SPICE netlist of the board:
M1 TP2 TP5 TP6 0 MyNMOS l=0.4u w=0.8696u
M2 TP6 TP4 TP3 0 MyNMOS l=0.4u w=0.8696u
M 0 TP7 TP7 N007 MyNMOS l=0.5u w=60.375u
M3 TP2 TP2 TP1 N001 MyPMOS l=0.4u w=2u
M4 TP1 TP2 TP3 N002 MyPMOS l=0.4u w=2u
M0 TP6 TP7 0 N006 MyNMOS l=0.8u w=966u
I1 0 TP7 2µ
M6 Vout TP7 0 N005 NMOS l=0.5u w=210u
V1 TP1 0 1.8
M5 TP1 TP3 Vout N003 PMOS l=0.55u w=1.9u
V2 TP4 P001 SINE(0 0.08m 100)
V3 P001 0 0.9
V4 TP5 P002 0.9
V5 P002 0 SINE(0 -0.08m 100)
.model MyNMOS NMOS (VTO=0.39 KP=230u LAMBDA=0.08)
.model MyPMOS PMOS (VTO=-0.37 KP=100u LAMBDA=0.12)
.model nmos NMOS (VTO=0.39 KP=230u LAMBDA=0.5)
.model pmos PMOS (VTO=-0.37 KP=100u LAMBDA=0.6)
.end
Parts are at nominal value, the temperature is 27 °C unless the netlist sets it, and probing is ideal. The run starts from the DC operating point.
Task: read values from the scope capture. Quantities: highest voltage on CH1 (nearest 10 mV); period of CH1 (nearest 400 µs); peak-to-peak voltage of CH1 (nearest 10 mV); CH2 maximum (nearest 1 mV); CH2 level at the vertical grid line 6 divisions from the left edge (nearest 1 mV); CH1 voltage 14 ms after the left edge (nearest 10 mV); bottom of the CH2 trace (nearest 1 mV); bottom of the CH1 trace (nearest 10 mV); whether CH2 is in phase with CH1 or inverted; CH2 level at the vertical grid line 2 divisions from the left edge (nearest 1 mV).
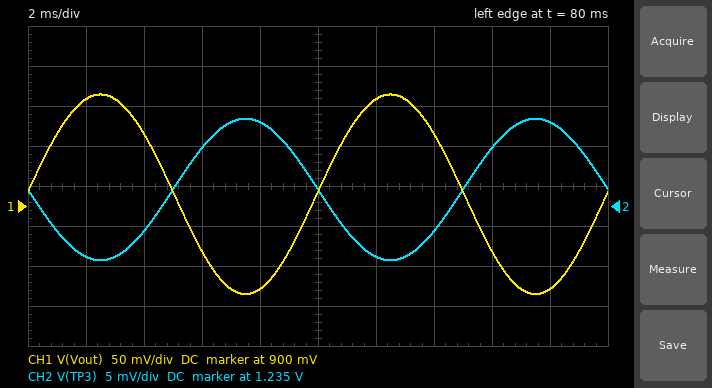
1.04 V
10.0 ms
250 mV
1.246 V
1.229 V
990 mV
1.228 V
790 mV
inverted
1.232 V
